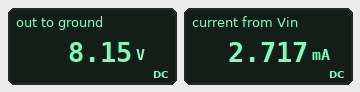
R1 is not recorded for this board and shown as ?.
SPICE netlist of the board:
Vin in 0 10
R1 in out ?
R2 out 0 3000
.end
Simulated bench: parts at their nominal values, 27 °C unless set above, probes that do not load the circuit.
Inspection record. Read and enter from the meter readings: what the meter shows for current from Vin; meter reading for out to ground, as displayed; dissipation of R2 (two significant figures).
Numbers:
2.717 mA
8.15 V
22 mW
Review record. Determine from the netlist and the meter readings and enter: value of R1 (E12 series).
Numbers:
680 Ω
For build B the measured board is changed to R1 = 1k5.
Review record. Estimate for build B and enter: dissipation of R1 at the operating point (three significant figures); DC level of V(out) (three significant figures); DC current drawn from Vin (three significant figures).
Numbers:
7.41 mW
6.67 V
2.22 mA
